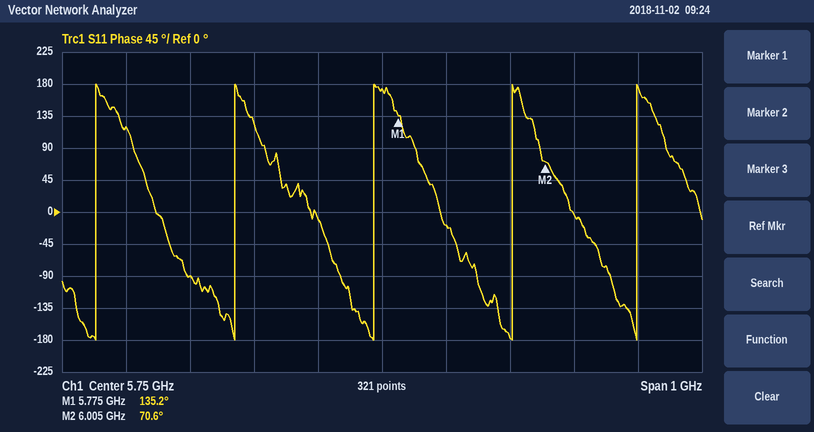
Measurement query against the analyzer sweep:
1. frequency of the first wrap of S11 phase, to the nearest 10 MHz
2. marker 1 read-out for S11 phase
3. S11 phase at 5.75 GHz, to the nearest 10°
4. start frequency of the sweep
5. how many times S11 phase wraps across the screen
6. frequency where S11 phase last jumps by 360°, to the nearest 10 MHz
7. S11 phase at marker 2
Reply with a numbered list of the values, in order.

1. 5.30 GHz
2. 135.2°
3. 170°
4. 5.25 GHz
5. 5
6. 6.15 GHz
7. 70.6°
